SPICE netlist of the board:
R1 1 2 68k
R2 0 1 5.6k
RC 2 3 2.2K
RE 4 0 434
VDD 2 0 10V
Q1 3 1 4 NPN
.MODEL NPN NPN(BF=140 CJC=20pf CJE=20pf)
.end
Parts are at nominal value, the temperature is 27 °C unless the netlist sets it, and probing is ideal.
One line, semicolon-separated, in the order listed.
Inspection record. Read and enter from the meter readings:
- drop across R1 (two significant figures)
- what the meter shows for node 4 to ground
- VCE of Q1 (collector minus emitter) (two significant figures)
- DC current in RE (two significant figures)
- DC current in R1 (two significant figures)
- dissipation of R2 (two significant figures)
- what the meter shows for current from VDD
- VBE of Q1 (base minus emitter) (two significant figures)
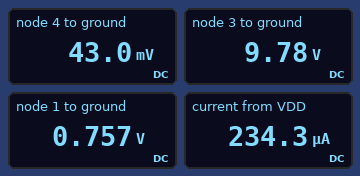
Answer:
9.2 V; 43.0 mV; 9.7 V; 99 µA; 140 µA; 100 µW; 234.3 µA; 710 mV
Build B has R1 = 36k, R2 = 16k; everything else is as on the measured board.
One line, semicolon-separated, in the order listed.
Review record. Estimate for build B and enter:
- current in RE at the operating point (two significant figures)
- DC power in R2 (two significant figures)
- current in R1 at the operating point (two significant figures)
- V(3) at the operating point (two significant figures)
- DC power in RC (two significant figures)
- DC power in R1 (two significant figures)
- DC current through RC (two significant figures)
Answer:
3.8 mA; 380 µW; 210 µA; 1.8 V; 31 mW; 1.6 mW; 3.7 mA
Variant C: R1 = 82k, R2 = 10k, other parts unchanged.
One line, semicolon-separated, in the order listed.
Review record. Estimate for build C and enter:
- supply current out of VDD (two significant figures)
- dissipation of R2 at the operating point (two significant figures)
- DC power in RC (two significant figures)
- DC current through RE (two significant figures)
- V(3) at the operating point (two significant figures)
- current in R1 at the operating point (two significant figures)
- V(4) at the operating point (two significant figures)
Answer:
760 µA; 110 µW; 920 µW; 650 µA; 8.6 V; 110 µA; 280 mV
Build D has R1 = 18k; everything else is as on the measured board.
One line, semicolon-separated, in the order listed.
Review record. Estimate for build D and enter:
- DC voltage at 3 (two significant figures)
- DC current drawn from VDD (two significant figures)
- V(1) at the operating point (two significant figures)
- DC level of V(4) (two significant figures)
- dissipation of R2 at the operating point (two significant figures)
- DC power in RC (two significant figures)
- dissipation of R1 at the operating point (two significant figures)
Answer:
2.6 V; 3.8 mA; 2.3 V; 1.5 V; 920 µW; 25 mW; 3.3 mW
